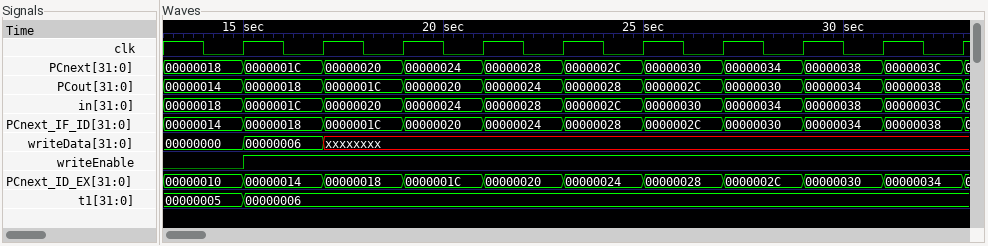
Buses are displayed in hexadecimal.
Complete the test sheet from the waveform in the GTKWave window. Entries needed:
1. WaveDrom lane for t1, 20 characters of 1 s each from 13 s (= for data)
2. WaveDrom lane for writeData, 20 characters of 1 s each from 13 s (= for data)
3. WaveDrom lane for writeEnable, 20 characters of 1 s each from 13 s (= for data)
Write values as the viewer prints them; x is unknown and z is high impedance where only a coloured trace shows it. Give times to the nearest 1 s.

{name: 't1', wave: '=.=.................', data: '00000005 00000006'}
{name: 'writeData', wave: '=.=.x...............', data: '00000000 00000006'}
{name: 'writeEnable', wave: '0.1.................'}
